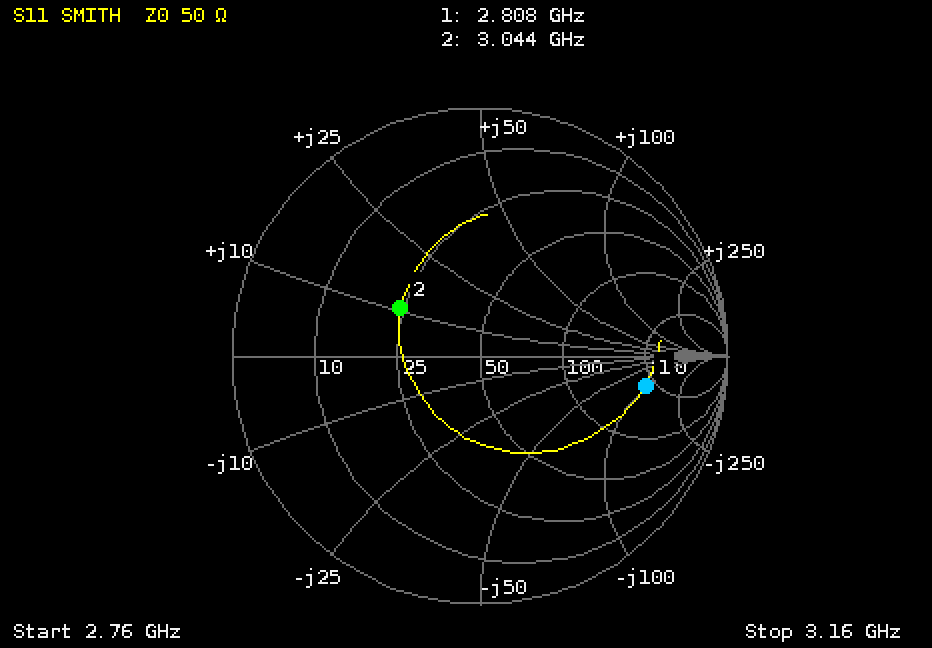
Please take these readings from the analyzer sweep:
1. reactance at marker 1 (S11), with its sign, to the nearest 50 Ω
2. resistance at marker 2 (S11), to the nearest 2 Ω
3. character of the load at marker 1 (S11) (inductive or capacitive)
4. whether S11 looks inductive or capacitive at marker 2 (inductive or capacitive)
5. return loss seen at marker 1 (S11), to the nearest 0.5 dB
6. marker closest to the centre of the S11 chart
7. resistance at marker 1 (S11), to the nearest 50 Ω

-100 Ω
24 Ω
capacitive
inductive
3.5 dB
marker 2
200 Ω
